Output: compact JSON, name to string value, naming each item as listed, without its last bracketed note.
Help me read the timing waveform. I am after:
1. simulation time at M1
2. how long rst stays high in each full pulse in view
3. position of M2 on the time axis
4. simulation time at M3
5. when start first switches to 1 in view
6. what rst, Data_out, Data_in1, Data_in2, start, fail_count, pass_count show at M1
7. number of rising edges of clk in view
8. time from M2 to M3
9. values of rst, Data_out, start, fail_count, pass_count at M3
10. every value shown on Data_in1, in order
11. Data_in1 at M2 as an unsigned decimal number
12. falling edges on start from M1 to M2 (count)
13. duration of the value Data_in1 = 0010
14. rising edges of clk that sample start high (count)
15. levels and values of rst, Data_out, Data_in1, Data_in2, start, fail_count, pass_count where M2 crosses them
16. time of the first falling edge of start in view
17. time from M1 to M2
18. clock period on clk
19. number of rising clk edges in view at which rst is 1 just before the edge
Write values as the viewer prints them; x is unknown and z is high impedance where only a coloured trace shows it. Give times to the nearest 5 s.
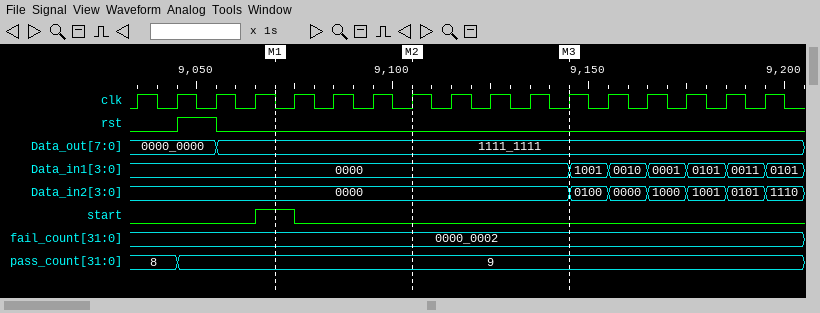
{"simulation time at M1": "9070 s", "how long rst stays high in each full pulse in view": "10 s", "position of M2 on the time axis": "9105 s", "simulation time at M3": "9145 s", "when start first switches to 1 in view": "9065 s", "what rst, Data_out, Data_in1, Data_in2, start, fail_count, pass_count show at M1": "rst=0, Data_out=1111_1111, Data_in1=0000, Data_in2=0000, start=1, fail_count=0000_0002, pass_count=9", "number of rising edges of clk in view": "17", "time from M2 to M3": "40 s", "values of rst, Data_out, start, fail_count, pass_count at M3": "rst=0, Data_out=1111_1111, start=0, fail_count=0000_0002, pass_count=9", "every value shown on Data_in1, in order": "0000, 1001, 0010, 0001, 0101, 0011, 0101", "Data_in1 at M2 as an unsigned decimal number": "0", "falling edges on start from M1 to M2": "1", "duration of the value Data_in1 = 0010": "10 s", "rising edges of clk that sample start high": "1", "levels and values of rst, Data_out, Data_in1, Data_in2, start, fail_count, pass_count where M2 crosses them": "rst=0, Data_out=1111_1111, Data_in1=0000, Data_in2=0000, start=0, fail_count=0000_0002, pass_count=9", "time of the first falling edge of start in view": "9075 s", "time from M1 to M2": "35 s", "clock period on clk": "10 s", "number of rising clk edges in view at which rst is 1 just before the edge": "1"}
